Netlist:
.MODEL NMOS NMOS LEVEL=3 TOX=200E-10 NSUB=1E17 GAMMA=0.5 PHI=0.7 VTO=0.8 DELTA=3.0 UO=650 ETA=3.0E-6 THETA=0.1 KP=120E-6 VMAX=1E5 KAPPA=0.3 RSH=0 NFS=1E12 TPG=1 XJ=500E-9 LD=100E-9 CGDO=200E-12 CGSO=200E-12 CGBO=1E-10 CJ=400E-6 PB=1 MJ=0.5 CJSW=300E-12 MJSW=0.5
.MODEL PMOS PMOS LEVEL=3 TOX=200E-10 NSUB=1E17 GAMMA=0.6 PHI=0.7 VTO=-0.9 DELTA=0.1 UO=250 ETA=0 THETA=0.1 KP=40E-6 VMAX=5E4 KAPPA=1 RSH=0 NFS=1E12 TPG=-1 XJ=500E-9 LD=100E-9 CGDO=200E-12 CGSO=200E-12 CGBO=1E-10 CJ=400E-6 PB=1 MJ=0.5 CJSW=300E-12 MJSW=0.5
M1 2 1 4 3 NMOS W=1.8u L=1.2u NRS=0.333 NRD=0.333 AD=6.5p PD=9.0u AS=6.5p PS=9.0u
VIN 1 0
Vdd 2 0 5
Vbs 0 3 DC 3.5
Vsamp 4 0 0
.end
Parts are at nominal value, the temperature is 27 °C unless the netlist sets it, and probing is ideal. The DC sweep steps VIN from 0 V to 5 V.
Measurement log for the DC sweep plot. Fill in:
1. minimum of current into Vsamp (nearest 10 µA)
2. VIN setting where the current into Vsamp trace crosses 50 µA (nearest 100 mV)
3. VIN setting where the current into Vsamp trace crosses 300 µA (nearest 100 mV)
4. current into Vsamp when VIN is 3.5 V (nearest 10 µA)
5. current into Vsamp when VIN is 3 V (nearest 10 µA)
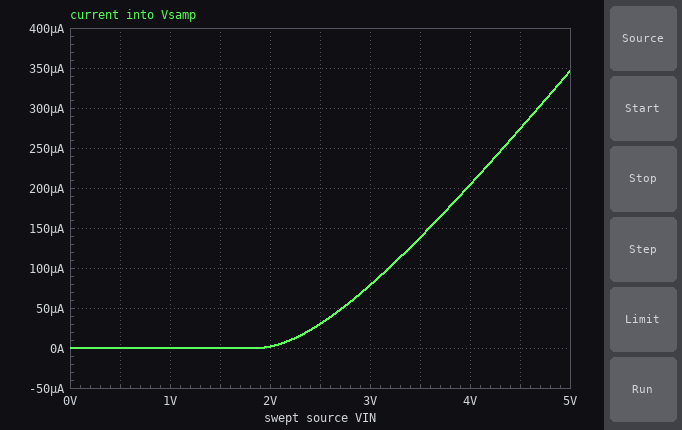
0 A
2.7 V
4.7 V
140 µA
80 µA
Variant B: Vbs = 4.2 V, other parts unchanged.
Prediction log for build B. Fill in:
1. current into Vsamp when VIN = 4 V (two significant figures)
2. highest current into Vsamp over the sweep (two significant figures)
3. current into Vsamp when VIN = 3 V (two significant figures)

180 µA
320 µA
61 µA
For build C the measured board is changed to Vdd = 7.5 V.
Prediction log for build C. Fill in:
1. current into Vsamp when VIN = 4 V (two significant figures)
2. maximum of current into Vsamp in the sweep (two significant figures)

210 µA
360 µA
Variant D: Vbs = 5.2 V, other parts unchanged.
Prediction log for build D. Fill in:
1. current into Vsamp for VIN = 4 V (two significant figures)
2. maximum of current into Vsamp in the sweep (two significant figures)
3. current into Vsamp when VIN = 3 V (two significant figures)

150 µA
290 µA
40 µA
